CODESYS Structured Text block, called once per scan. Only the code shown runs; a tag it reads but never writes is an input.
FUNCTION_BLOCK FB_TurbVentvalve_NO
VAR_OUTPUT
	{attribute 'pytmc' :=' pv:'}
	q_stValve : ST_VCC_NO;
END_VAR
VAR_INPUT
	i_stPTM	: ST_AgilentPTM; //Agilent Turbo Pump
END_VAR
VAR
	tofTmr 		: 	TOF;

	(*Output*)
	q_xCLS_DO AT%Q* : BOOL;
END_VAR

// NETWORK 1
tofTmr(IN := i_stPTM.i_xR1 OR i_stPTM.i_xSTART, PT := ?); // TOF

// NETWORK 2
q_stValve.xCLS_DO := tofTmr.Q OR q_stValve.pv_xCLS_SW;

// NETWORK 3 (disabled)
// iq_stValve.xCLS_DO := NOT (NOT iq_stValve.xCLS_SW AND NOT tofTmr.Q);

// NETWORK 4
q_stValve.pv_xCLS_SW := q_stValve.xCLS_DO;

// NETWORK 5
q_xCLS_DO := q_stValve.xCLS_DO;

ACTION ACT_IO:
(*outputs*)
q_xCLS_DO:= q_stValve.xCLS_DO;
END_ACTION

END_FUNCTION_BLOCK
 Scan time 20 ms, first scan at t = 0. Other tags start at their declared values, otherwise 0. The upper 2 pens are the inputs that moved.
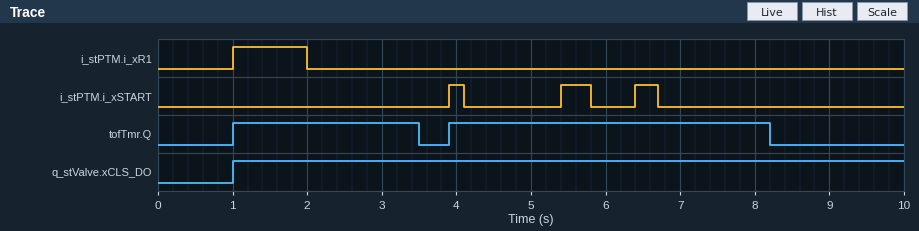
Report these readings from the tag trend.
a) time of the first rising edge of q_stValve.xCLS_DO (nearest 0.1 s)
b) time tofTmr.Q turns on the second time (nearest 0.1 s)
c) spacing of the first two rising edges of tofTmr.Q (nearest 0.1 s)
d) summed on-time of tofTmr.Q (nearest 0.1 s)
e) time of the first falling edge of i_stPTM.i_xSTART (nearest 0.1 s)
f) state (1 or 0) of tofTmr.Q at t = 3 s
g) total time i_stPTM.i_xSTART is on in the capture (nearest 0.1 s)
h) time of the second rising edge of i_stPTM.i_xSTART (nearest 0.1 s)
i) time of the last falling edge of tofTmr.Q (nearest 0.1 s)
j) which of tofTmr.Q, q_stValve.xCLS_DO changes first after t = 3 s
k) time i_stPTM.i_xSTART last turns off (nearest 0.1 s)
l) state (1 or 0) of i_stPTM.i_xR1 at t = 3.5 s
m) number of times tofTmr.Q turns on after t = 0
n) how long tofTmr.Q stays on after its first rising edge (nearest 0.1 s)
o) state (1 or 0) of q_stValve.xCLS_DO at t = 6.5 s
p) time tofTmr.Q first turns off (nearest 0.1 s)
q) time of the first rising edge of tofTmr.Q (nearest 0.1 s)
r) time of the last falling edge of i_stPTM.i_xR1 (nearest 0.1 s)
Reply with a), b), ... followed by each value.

a) 1.0 s
b) 3.9 s
c) 2.9 s
d) 6.8 s
e) 4.1 s
f) 1
g) 0.9 s
h) 5.4 s
i) 8.2 s
j) tofTmr.Q
k) 6.7 s
l) 0
m) 2
n) 2.5 s
o) 1
p) 3.5 s
q) 1.0 s
r) 2.0 s
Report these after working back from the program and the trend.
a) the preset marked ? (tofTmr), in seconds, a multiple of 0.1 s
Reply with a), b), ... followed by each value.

a) 1.5 s
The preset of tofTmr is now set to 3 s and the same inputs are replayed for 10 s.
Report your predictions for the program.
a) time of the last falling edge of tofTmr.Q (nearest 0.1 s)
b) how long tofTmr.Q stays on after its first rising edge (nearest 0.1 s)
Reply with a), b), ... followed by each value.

a) 9.7 s
b) 8.7 s
